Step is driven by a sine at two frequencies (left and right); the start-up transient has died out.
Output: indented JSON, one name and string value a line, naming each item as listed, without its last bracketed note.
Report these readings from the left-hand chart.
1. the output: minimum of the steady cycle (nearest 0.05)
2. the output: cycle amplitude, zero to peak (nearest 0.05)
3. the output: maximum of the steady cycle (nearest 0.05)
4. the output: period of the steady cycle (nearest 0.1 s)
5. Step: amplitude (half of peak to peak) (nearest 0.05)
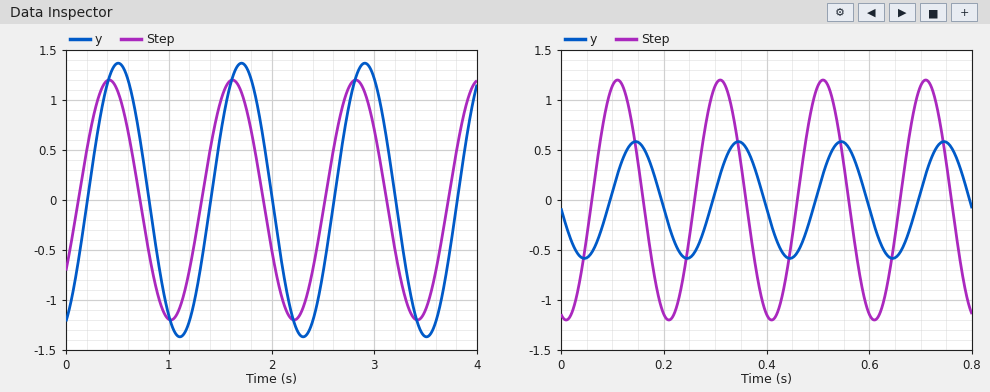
{
  "the output: minimum of the steady cycle": "-1.35",
  "the output: cycle amplitude, zero to peak": "1.35",
  "the output: maximum of the steady cycle": "1.35",
  "the output: period of the steady cycle": "1.2 s",
  "Step: amplitude (half of peak to peak)": "1.20"
}
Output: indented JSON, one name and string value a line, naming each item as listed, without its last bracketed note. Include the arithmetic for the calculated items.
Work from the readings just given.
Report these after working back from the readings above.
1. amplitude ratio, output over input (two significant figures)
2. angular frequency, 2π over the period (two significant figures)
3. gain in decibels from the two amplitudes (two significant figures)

{
  "amplitude ratio, output over input": "1.35 / 1.2 = 1.1",
  "angular frequency, 2π over the period": "2π / 1.2 = 5.2 rad/s",
  "gain in decibels from the two amplitudes": "20 log10(1.35 / 1.2) = 1.0 dB"
}
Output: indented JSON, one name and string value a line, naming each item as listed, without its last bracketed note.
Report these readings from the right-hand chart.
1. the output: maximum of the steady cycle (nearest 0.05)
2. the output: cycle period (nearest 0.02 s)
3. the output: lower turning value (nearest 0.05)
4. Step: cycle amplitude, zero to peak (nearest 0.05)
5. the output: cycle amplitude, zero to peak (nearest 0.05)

{
  "the output: maximum of the steady cycle": "0.60",
  "the output: cycle period": "0.20 s",
  "the output: lower turning value": "-0.60",
  "Step: cycle amplitude, zero to peak": "1.20",
  "the output: cycle amplitude, zero to peak": "0.60"
}
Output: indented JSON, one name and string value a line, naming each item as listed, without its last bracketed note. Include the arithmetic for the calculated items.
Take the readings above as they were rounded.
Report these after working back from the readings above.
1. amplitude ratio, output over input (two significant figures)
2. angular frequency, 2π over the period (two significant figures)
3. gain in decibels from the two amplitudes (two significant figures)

{
  "amplitude ratio, output over input": "0.6 / 1.2 = 0.50",
  "angular frequency, 2π over the period": "2π / 0.2 = 31 rad/s",
  "gain in decibels from the two amplitudes": "20 log10(0.6 / 1.2) = -6.0 dB"
}
